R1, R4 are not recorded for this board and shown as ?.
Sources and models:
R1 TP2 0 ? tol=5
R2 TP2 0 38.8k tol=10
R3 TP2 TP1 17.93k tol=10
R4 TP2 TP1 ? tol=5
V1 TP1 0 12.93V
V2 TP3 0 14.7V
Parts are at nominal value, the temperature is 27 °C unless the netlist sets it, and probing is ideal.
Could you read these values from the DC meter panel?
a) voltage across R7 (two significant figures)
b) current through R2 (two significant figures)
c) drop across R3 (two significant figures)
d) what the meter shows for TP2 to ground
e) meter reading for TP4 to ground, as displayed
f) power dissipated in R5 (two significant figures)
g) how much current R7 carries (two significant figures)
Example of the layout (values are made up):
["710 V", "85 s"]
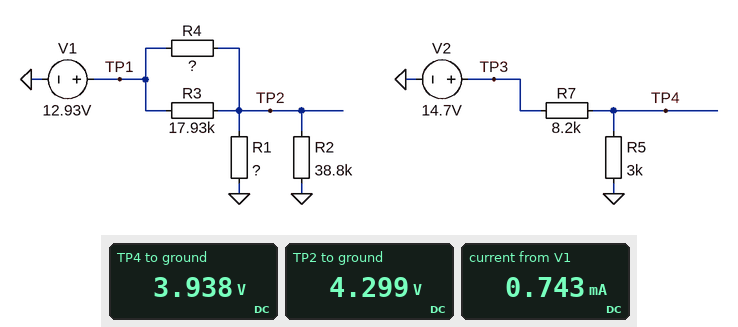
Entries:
["11 V", "110 µA", "8.6 V", "4.299 V", "3.938 V", "5.2 mW", "1.3 mA"]
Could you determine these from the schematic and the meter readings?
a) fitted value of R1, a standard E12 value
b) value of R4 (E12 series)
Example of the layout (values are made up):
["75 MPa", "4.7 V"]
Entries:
["6.8 kΩ", "33 kΩ"]
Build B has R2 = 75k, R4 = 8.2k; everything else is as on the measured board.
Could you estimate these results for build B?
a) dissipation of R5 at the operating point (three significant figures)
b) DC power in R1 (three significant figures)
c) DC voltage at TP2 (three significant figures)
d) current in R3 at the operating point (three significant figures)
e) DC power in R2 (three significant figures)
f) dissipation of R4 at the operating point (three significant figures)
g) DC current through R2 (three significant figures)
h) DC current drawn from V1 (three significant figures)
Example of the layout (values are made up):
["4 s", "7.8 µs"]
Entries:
["5.17 mW", "6.79 mW", "6.80 V", "342 µA", "616 µW", "4.59 mW", "90.6 µA", "1.09 mA"]
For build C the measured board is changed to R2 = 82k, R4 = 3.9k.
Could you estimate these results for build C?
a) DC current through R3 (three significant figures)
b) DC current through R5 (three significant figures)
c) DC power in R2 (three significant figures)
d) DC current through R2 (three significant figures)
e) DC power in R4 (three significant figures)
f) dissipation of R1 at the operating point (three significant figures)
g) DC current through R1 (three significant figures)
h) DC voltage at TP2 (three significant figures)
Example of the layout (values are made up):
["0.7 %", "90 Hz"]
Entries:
["244 µA", "1.31 mA", "894 µW", "104 µA", "4.89 mW", "10.8 mW", "1.26 mA", "8.56 V"]
